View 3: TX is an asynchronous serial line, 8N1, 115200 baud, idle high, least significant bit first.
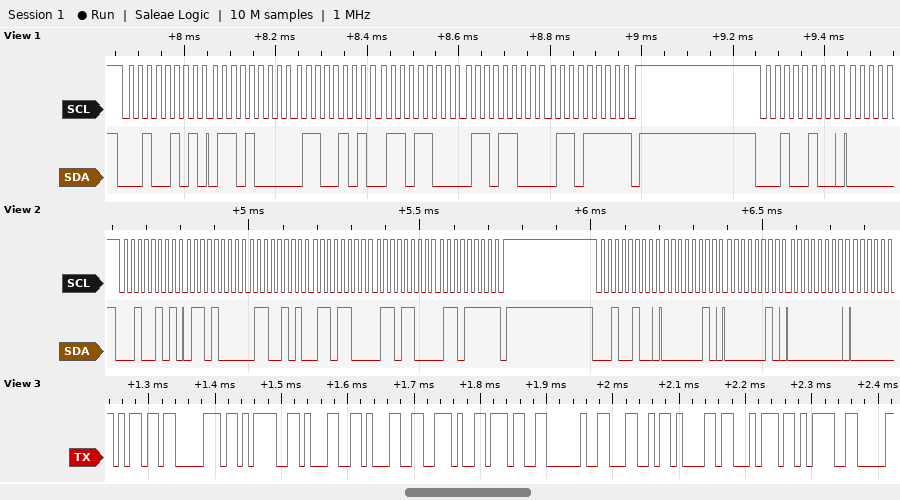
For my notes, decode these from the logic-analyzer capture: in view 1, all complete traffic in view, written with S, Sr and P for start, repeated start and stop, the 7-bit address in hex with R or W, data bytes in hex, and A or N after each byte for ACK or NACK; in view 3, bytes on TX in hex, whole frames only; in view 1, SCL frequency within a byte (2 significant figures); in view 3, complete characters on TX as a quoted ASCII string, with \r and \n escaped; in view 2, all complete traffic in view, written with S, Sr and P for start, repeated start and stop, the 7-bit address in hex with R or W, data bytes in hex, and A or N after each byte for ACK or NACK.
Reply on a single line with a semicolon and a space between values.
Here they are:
S 12R A 68 A 65 A 6C A 6C A 6F N P S 12W A; 6D 70 3D 31 31 2E 37 20 4C 61 74 3D; 50 kHz; "mp=11.7 Lat="; S 12R A 68 A 65 A 6C A 6C A 6F N P S 12W A 02 A 02 A 00 A
